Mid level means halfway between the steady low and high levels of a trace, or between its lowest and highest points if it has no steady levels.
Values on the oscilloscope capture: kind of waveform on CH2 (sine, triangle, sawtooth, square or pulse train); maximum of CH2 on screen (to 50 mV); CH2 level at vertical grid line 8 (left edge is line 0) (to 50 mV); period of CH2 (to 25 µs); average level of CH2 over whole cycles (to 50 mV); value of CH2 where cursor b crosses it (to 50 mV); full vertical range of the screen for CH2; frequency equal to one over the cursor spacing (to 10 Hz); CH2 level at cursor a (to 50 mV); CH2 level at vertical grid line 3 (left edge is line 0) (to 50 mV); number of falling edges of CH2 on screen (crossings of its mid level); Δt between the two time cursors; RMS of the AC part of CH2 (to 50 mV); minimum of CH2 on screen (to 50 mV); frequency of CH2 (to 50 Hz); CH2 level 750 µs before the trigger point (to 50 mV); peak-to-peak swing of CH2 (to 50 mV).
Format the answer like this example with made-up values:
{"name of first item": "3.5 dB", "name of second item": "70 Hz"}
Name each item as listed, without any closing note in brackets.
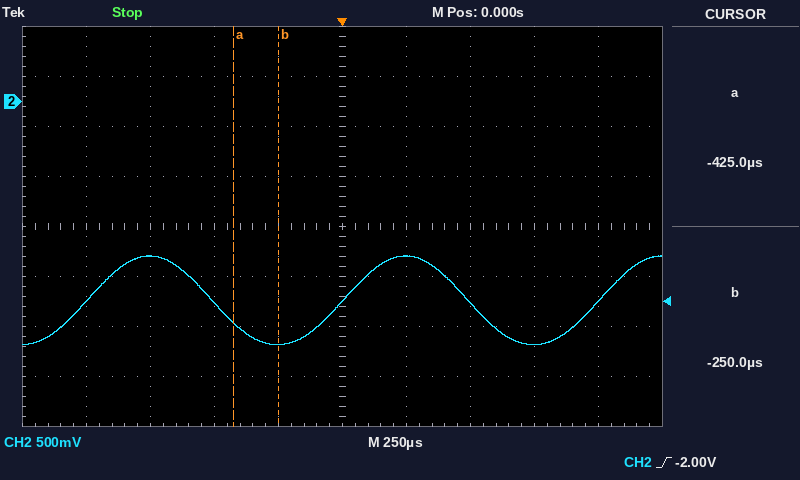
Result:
{"kind of waveform on CH2": "sine", "maximum of CH2 on screen": "-1.55 V", "CH2 level at vertical grid line 8 (left edge is line 0)": "-2.45 V", "period of CH2": "1.000 ms", "average level of CH2 over whole cycles": "-2.00 V", "value of CH2 where cursor b crosses it": "-2.45 V", "full vertical range of the screen for CH2": "4 V", "frequency equal to one over the cursor spacing": "5.71 kHz", "CH2 level at cursor a": "-2.20 V", "CH2 level at vertical grid line 3 (left edge is line 0)": "-2.00 V", "number of falling edges of CH2 on screen": "2", "Δt between the two time cursors": "175 µs", "RMS of the AC part of CH2": "300 mV", "minimum of CH2 on screen": "-2.45 V", "frequency of CH2": "1.00 kHz", "CH2 level 750 µs before the trigger point": "-1.55 V", "peak-to-peak swing of CH2": "900 mV"}
